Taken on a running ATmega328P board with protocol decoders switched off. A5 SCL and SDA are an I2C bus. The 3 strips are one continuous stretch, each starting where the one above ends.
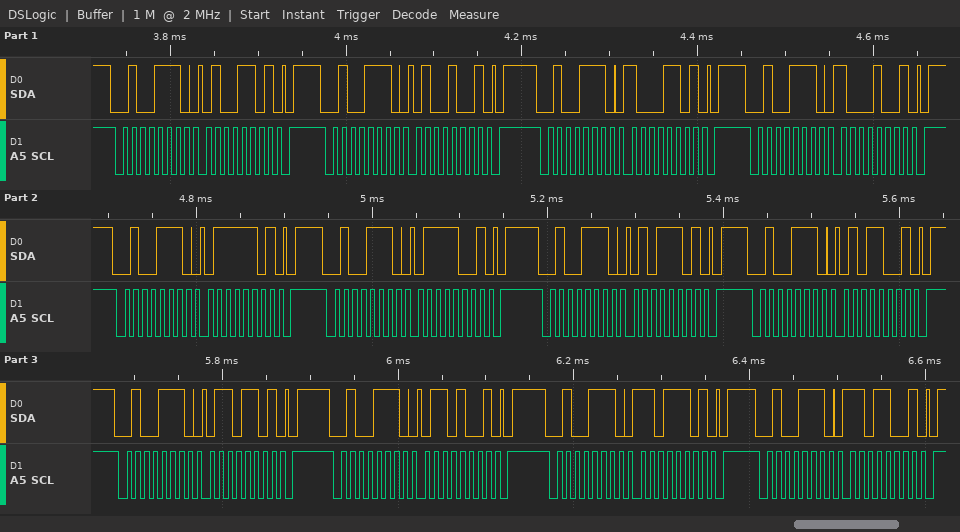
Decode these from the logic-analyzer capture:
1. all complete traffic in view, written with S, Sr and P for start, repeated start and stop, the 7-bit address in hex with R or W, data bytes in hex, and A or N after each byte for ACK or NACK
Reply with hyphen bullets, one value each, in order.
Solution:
- S 27W A 4D A P S 27W A 49 A P S 27W A 8D A P S 27W A 89 A P S 27W A 7D A P S 27W A 79 A P S 27W A 5D A P S 27W A 59 A P S 27W A 6D A P S 27W A 69 A P S 27W A DD A P S 27W A D9 A P
